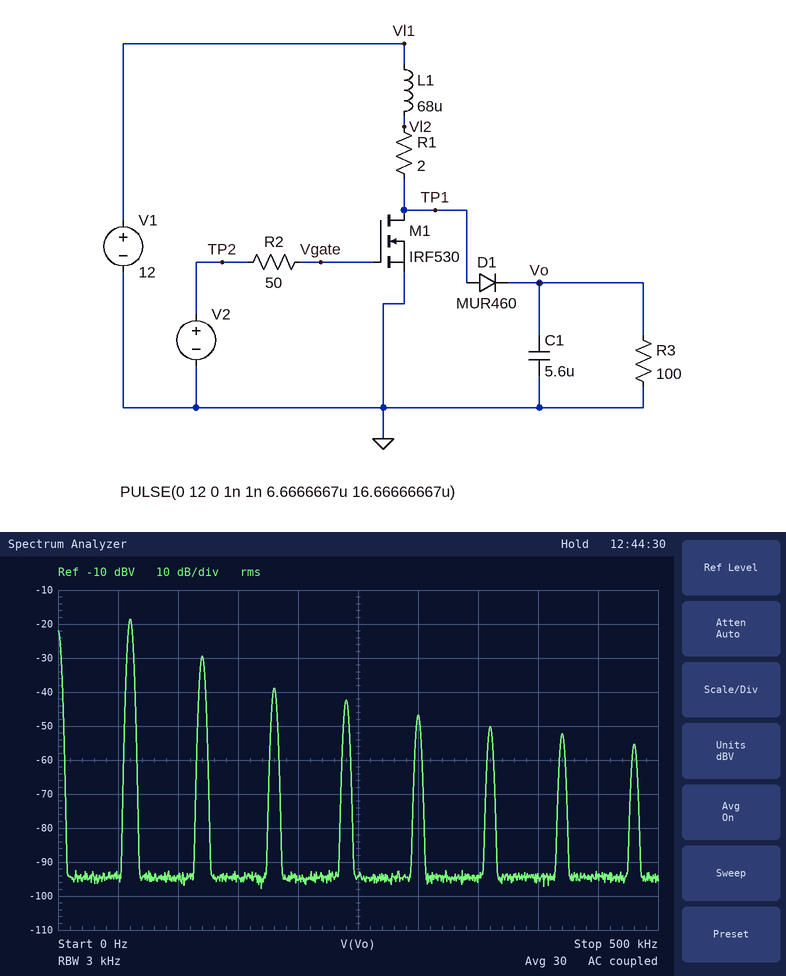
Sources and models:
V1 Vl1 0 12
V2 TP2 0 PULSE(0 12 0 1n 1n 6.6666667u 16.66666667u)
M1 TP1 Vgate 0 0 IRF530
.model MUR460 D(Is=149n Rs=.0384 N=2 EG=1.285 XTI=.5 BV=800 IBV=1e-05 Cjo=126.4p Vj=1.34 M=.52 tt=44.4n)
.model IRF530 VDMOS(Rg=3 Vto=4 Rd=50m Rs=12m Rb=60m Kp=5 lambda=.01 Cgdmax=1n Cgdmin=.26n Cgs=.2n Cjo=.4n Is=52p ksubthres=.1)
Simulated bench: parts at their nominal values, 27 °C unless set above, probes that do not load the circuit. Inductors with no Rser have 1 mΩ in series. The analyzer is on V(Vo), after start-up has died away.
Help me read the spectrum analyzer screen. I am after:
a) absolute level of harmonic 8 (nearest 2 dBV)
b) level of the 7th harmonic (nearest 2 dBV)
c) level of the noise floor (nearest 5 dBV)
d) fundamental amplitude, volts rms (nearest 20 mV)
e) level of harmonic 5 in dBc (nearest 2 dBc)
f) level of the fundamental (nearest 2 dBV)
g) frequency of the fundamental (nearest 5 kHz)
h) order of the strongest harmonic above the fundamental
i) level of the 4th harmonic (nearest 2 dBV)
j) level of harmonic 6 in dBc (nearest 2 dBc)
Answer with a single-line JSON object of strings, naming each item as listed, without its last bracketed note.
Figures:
{"absolute level of harmonic 8": "-56 dBV", "level of the 7th harmonic": "-52 dBV", "level of the noise floor": "-95 dBV", "fundamental amplitude, volts rms": "120 mV", "level of harmonic 5 in dBc": "-28 dBc", "level of the fundamental": "-18 dBV", "frequency of the fundamental": "60 kHz", "order of the strongest harmonic above the fundamental": "2", "level of the 4th harmonic": "-42 dBV", "level of harmonic 6 in dBc": "-32 dBc"}
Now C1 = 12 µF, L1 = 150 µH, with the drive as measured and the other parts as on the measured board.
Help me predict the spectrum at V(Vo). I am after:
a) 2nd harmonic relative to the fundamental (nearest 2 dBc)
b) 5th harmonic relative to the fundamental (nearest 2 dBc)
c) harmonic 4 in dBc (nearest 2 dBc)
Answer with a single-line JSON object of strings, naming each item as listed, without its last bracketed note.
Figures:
{"2nd harmonic relative to the fundamental": "-16 dBc", "5th harmonic relative to the fundamental": "-30 dBc", "harmonic 4 in dBc": "-26 dBc"}
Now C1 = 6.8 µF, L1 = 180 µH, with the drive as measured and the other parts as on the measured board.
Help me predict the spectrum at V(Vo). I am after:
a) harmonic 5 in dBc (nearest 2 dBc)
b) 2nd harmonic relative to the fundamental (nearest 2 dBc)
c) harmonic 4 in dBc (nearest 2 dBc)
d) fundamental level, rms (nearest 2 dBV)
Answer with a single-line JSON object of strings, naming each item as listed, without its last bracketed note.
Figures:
{"harmonic 5 in dBc": "-32 dBc", "2nd harmonic relative to the fundamental": "-16 dBc", "harmonic 4 in dBc": "-26 dBc", "fundamental level, rms": "-24 dBV"}
